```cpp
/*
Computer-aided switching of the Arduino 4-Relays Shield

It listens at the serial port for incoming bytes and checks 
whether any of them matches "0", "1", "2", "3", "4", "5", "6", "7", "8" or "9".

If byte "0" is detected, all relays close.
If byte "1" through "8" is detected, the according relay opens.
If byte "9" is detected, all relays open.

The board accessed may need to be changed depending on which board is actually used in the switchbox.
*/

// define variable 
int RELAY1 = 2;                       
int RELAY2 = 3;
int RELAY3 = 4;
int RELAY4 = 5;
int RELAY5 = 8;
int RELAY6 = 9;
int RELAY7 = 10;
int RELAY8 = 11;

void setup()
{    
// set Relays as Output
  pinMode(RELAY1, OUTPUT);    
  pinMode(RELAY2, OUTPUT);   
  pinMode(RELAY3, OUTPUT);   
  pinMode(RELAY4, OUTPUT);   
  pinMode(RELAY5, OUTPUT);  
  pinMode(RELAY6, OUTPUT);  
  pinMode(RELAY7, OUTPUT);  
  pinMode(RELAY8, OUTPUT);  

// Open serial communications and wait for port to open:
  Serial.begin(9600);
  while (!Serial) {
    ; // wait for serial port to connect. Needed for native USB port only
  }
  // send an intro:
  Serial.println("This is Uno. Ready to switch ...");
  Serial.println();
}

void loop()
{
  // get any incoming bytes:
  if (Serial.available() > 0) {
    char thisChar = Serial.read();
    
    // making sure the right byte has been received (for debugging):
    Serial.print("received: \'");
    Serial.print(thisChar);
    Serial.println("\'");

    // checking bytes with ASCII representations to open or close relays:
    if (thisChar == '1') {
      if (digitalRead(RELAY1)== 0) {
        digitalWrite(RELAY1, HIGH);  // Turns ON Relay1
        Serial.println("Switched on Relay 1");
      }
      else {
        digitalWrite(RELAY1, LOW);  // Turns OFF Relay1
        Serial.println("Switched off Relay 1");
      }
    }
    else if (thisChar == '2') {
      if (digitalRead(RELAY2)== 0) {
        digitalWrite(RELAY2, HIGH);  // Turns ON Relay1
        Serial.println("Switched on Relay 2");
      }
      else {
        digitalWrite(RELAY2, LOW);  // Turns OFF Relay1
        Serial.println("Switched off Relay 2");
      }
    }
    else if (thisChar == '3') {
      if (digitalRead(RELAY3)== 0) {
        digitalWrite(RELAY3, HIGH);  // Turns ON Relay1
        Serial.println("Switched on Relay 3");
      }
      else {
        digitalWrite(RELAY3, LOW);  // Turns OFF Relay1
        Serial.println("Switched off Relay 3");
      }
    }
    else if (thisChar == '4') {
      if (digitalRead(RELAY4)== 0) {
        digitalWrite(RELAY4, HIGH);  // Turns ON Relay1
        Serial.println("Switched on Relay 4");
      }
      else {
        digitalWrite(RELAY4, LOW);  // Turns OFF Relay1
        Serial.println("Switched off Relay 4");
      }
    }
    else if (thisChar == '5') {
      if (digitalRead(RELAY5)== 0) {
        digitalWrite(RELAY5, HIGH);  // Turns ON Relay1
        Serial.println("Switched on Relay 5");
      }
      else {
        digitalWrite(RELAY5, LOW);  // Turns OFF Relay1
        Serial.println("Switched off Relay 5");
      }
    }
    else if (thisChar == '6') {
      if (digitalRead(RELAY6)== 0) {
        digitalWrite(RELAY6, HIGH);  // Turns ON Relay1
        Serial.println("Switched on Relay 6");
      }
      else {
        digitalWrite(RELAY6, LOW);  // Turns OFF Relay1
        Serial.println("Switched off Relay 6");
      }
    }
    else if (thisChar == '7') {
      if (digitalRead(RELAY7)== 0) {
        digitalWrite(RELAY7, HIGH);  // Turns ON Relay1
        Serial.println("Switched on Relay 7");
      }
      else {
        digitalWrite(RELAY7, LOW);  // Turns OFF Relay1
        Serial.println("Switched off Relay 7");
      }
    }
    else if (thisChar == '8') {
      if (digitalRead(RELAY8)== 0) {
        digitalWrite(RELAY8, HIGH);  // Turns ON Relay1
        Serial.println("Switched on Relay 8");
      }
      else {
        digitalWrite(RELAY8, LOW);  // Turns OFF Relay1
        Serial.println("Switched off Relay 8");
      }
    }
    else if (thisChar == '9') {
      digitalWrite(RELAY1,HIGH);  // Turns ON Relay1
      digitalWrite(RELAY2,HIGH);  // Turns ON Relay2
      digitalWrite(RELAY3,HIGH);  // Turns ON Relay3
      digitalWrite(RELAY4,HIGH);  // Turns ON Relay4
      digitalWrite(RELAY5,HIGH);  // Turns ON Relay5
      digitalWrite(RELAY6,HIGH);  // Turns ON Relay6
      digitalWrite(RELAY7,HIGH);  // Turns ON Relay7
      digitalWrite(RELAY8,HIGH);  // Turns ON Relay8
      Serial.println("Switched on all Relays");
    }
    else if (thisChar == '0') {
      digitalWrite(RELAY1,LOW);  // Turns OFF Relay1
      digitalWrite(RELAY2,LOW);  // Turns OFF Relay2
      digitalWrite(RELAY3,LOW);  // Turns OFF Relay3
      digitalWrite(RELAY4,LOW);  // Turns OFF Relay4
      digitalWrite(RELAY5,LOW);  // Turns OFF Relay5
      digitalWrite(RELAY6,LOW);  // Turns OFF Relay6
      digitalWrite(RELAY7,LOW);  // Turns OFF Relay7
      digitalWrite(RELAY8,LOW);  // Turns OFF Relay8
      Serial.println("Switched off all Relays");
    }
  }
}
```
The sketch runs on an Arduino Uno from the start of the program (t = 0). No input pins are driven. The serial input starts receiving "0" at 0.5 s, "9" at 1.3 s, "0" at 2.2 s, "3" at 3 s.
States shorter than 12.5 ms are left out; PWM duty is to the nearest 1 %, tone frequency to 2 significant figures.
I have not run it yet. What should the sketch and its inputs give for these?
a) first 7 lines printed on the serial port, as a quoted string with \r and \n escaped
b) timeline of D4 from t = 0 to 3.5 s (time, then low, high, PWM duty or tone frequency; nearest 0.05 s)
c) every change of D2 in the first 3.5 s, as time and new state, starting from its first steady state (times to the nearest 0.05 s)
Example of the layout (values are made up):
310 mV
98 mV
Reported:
"This is Uno. Ready to switch ...\r\n\r\nreceived: '0'\r\nSwitched off all Relays\r\nreceived: '9'\r\nSwitched on all Relays\r\nreceived: '0'\r\n"
0 s low; 1.3 s high; 2.2 s low; 3 s high
0 s low; 1.3 s high; 2.2 s low
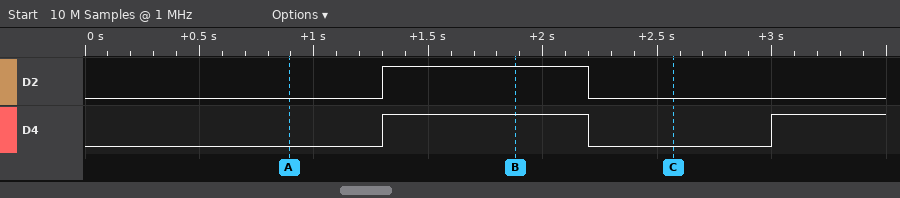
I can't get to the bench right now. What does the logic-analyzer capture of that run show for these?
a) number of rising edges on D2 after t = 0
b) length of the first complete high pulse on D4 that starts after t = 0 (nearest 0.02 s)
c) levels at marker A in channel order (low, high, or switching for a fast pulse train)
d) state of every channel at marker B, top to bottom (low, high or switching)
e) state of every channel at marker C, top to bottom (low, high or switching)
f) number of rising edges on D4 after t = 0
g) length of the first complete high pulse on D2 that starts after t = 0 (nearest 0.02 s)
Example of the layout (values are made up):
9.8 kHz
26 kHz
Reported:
1
0.90 s
D2 low, D4 low
D2 high, D4 high
D2 low, D4 low
2
0.90 s
